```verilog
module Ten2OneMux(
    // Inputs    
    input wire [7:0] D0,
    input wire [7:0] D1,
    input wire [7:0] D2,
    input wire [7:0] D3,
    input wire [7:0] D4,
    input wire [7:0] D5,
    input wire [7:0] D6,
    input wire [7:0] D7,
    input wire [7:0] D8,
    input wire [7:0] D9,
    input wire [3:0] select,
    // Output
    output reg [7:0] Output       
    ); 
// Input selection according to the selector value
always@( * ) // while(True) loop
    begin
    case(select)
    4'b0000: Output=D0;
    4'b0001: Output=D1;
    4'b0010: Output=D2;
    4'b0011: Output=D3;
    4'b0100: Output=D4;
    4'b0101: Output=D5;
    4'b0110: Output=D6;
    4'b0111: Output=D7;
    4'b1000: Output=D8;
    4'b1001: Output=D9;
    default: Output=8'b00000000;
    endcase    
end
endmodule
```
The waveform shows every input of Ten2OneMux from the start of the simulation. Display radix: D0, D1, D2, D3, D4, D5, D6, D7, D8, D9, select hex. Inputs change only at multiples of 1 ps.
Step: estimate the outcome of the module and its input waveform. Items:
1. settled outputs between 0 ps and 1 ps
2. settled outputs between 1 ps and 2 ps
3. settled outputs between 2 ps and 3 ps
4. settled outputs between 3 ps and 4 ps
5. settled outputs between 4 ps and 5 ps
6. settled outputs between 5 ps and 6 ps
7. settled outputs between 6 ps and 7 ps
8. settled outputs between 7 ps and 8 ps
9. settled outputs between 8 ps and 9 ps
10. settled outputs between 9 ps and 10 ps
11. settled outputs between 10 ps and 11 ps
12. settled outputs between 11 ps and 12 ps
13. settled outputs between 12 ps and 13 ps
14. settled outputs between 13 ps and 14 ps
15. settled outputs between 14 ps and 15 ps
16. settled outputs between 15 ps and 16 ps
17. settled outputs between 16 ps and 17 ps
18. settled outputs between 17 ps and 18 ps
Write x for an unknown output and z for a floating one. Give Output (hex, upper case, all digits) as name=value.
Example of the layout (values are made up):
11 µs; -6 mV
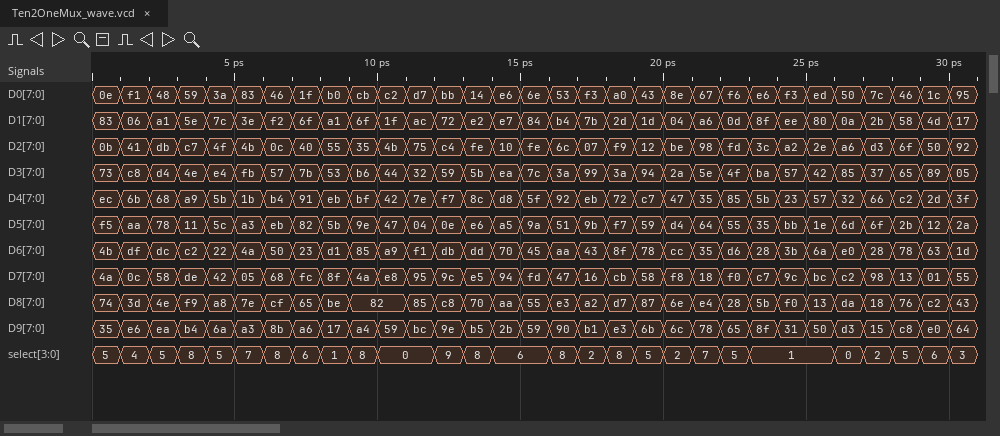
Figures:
Output=F5; Output=6B; Output=78; Output=F9; Output=5C; Output=05; Output=CF; Output=23; Output=A1; Output=82; Output=C2; Output=D7; Output=9E; Output=70; Output=70; Output=45; Output=E3; Output=07
